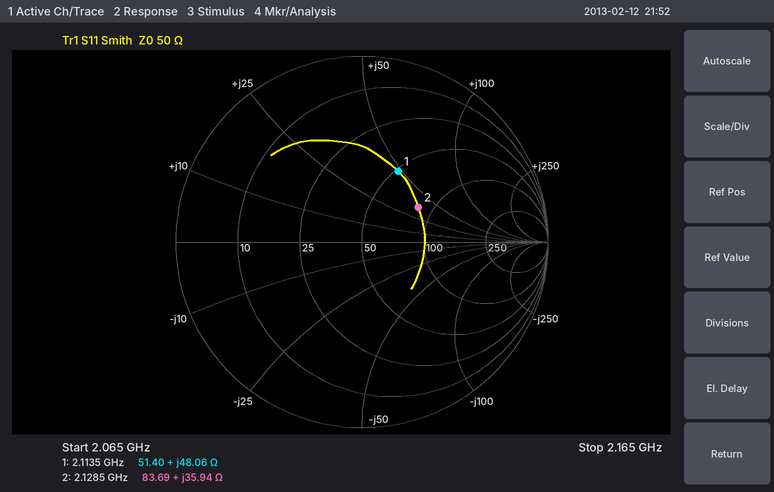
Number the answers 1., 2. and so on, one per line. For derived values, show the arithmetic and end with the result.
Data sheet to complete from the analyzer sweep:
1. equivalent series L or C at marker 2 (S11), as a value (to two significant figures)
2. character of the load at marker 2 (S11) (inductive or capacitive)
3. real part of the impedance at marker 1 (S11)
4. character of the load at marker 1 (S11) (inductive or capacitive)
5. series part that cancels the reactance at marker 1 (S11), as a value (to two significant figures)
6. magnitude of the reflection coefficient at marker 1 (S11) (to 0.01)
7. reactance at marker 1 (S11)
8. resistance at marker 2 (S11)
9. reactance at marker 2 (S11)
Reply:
1. L = 35.94 Ω/(2π × 2.1285 GHz) ≈ 2.7 nH
2. inductive
3. 51.40 Ω
4. inductive
5. C = 1/(2π × 2.1135 GHz × 48.06 Ω) ≈ 1.6 pF
6. 0.43
7. +48.06 Ω
8. 83.69 Ω
9. +35.94 Ω
